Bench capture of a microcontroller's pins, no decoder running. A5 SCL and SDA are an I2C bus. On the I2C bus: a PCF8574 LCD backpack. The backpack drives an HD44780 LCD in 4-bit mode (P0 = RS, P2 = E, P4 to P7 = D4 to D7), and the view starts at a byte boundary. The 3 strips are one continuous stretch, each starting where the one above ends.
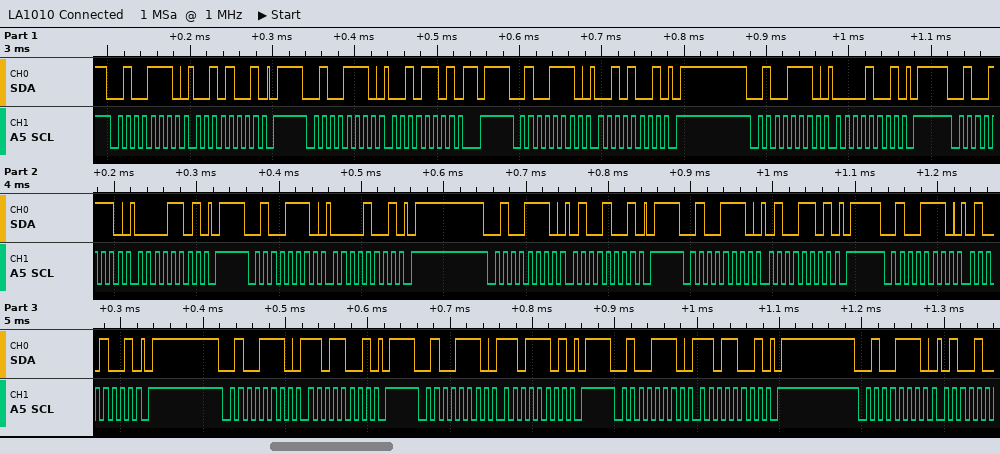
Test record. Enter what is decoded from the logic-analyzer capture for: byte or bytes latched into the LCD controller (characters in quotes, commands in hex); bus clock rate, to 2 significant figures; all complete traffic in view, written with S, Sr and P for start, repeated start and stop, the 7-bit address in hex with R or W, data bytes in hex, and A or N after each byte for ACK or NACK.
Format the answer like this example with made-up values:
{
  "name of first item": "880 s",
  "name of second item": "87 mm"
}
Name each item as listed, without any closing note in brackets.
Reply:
{
  "byte or bytes latched into the LCD controller": "' ' 'M'",
  "bus clock rate, to 2 significant figures": "100 kHz",
  "all complete traffic in view, written with S, Sr and P for start, repeated start and stop, the 7-bit address in hex with R or W, data bytes in hex, and A or N after each byte for ACK or NACK": "S 27W A 29 A P S 27W A 2D A P S 27W A 29 A P S 27W A 09 A P S 27W A 0D A P S 27W A 09 A P S 27W A 49 A P S 27W A 4D A P S 27W A 49 A P S 27W A D9 A P S 27W A DD A P S 27W A D9 A P S 27W A"
}
